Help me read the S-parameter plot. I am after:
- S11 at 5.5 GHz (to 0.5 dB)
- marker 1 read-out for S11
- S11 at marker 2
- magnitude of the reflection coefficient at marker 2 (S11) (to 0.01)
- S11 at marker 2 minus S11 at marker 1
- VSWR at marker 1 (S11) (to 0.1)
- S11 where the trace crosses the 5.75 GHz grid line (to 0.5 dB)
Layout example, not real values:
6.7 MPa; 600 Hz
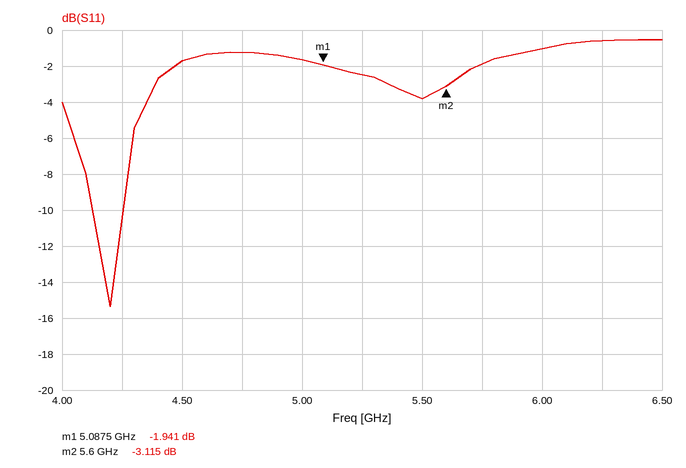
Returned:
-4.0 dB; -1.941 dB; -3.115 dB; 0.70; -1.174 dB; 9.0; -2.0 dB
